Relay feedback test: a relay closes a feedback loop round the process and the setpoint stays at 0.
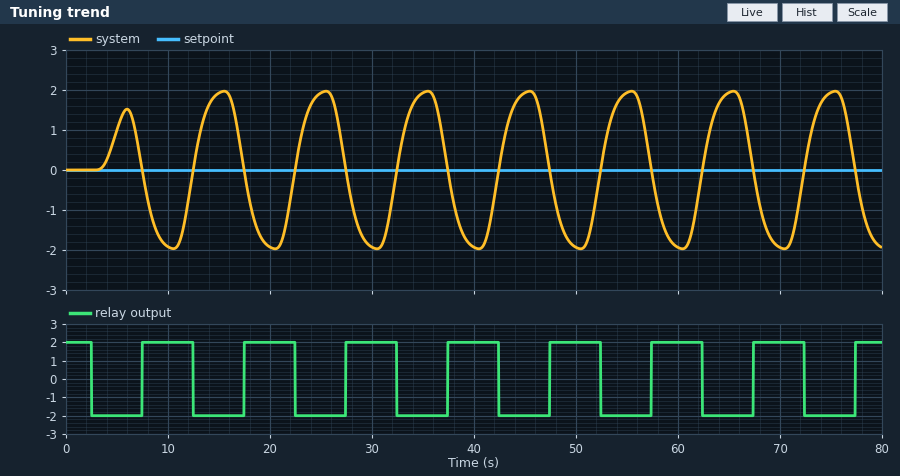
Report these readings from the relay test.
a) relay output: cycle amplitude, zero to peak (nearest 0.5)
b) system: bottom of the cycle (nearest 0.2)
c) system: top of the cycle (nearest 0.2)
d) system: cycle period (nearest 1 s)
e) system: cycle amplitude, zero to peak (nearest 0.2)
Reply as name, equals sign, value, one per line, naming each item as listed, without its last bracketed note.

relay output: cycle amplitude, zero to peak = 2.0
system: bottom of the cycle = -2.0
system: top of the cycle = 2.0
system: cycle period = 10 s
system: cycle amplitude, zero to peak = 2.0
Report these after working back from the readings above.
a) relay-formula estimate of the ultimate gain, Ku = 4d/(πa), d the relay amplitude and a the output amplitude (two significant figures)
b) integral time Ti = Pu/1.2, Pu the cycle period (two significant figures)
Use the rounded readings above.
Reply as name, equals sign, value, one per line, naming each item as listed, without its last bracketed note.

relay-formula estimate of the ultimate gain, Ku = 4d/(πa), d the relay amplitude and a the output amplitude = 1.3
integral time Ti = Pu/1.2, Pu the cycle period = 8.3 s
